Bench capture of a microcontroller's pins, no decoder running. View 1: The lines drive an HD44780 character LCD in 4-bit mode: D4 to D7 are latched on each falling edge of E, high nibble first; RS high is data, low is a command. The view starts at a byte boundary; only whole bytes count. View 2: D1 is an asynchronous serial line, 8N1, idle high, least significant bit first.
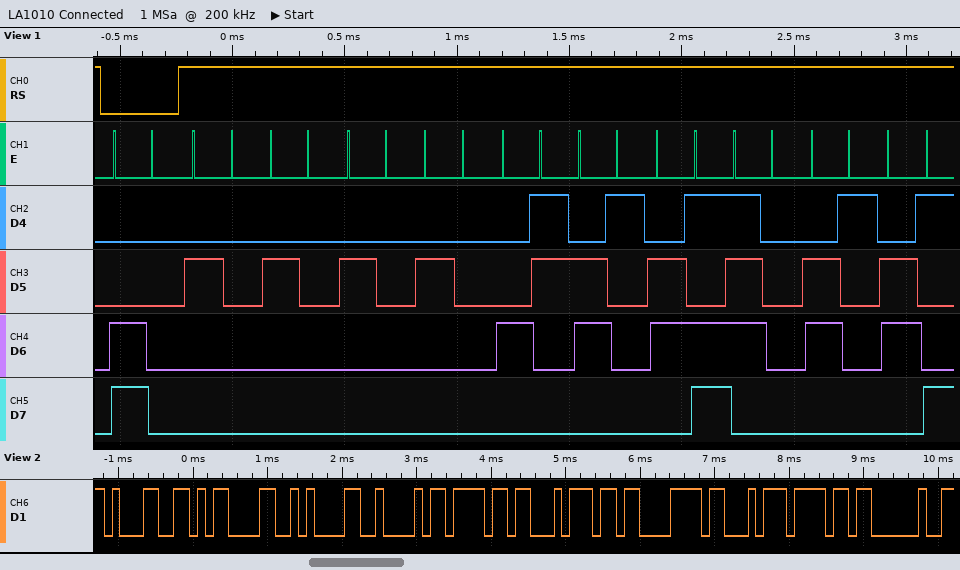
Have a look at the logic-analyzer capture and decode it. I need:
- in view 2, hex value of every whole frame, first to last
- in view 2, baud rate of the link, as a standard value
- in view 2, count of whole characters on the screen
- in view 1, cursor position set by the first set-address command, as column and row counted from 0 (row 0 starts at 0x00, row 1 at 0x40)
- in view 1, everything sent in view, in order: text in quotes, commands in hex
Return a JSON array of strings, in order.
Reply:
["31 0D 0A 42 6F 74 C3 A3 6F 20", "9600 baud", "10", "column 0, row 1", "0xC0 \"    Campai\""]
